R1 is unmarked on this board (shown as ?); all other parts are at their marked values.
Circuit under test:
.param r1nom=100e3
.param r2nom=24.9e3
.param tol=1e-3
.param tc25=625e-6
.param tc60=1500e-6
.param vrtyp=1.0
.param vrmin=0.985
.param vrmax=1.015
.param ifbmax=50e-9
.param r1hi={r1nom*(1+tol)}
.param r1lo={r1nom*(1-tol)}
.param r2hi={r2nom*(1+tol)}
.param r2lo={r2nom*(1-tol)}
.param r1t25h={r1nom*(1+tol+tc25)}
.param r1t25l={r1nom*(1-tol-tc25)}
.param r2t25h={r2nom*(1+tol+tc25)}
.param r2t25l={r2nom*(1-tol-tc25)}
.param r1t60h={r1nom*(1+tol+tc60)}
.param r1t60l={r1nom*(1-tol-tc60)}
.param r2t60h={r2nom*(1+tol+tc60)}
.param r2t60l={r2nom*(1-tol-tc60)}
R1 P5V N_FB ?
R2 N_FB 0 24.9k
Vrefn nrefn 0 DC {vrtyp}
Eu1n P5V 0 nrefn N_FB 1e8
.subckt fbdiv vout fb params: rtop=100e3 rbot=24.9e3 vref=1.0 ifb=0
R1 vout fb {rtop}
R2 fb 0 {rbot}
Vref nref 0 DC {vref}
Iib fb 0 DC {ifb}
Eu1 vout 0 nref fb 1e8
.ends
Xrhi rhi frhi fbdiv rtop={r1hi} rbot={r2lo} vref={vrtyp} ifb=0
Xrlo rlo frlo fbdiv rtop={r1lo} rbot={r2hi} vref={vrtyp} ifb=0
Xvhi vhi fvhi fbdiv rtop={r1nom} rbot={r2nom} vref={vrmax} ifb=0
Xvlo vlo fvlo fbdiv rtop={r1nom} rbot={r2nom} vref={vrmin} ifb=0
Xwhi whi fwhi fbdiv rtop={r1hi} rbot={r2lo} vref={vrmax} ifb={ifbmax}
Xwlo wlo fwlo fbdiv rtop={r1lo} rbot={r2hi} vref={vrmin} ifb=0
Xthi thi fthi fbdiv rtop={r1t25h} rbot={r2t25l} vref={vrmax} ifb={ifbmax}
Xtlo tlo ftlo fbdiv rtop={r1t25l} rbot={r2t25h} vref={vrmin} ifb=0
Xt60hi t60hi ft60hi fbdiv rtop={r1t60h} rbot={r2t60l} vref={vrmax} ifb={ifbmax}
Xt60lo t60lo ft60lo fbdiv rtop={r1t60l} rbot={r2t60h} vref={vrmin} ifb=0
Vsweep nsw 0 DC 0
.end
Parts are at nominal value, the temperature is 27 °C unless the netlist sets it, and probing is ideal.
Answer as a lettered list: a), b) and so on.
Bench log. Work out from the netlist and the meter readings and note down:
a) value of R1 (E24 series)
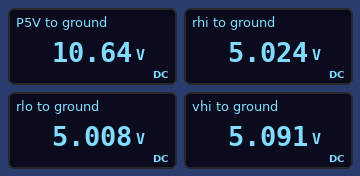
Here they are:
a) 240 kΩ
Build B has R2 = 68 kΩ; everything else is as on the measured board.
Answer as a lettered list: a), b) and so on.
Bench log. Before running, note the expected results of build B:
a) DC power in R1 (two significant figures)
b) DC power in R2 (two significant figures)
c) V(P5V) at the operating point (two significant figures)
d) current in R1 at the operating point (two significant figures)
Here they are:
a) 52 µW
b) 15 µW
c) 4.5 V
d) 15 µA
